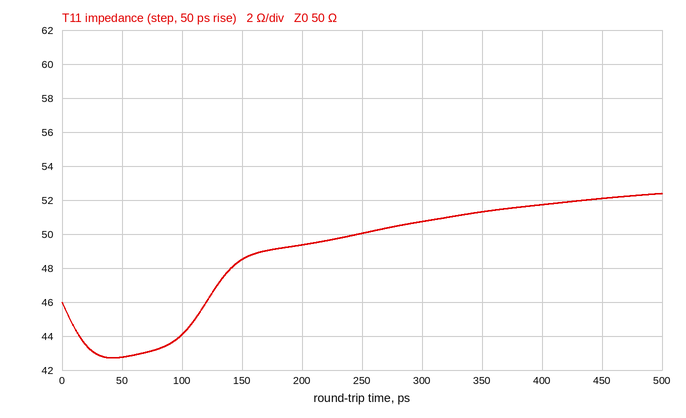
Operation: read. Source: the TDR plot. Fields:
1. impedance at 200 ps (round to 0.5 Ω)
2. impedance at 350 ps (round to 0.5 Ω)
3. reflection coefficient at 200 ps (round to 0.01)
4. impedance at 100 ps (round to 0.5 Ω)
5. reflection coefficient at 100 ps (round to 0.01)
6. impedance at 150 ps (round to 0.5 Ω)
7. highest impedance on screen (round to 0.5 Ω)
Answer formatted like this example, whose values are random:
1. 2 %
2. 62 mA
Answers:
1. 49.5 Ω
2. 51.5 Ω
3. -0.01
4. 44.0 Ω
5. -0.06
6. 48.5 Ω
7. 52.5 Ω
